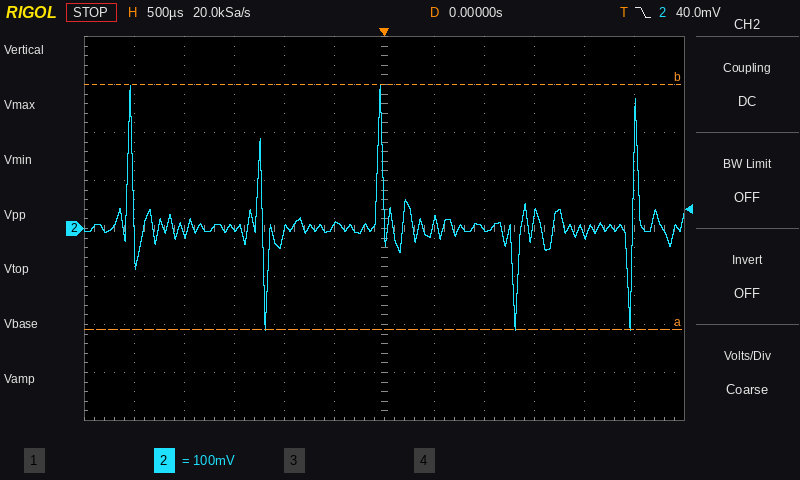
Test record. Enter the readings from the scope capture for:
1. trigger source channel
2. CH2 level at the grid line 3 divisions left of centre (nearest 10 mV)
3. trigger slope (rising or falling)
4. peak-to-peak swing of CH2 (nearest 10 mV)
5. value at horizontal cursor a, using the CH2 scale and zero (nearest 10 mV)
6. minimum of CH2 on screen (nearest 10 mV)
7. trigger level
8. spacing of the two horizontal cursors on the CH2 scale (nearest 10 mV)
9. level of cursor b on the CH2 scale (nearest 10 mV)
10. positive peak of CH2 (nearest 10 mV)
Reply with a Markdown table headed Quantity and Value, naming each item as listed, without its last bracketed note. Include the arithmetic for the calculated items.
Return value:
| Quantity | Value |
|---|---|
| trigger source channel | CH2 |
| CH2 level at the grid line 3 divisions left of centre | 0 mV |
| trigger slope | falling |
| peak-to-peak swing of CH2 | 300 mV − (-210 mV) = 510 mV |
| value at horizontal cursor a, using the CH2 scale and zero | -210 mV |
| minimum of CH2 on screen | -210 mV |
| trigger level | 40.0 mV |
| spacing of the two horizontal cursors on the CH2 scale | 510 mV |
| level of cursor b on the CH2 scale | 300 mV |
| positive peak of CH2 | 300 mV |
